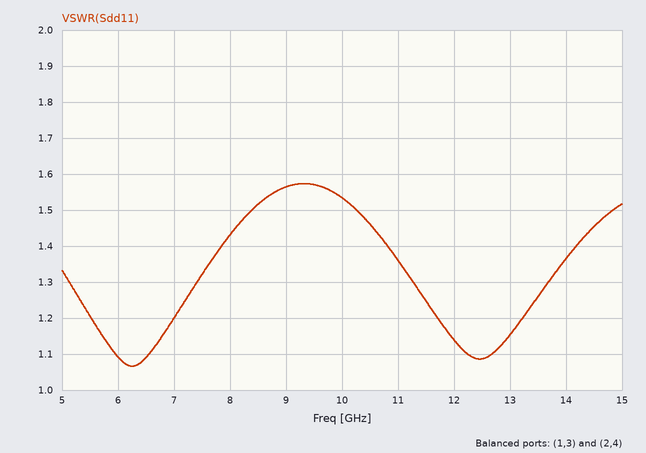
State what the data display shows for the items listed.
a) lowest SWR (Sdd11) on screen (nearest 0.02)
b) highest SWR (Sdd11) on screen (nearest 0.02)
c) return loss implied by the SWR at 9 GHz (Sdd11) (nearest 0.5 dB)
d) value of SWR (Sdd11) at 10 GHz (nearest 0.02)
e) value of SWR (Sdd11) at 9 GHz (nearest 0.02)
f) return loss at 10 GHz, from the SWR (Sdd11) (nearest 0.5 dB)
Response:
1.06
1.58
13.0 dB
1.54
1.56
13.5 dB
